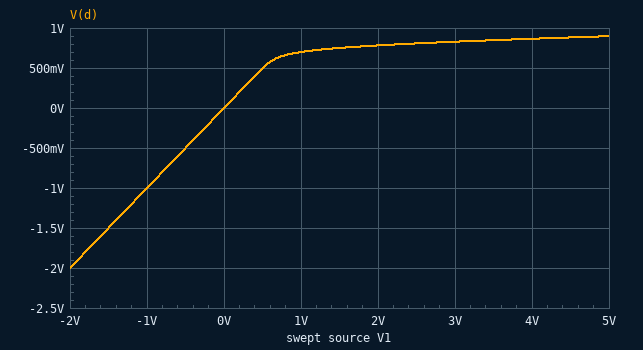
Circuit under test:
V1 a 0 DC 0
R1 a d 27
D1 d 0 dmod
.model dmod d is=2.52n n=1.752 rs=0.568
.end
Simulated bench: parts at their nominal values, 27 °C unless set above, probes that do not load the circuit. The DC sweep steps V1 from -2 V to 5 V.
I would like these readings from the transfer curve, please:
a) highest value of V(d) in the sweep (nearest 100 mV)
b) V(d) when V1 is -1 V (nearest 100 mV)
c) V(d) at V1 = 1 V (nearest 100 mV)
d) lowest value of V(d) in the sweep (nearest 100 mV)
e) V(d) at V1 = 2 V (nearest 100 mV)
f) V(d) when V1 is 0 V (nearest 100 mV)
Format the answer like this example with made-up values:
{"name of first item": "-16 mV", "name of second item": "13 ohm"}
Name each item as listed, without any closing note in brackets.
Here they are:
{"highest value of V(d) in the sweep": "900 mV", "V(d) when V1 is -1 V": "-1.0 V", "V(d) at V1 = 1 V": "700 mV", "lowest value of V(d) in the sweep": "-2.0 V", "V(d) at V1 = 2 V": "800 mV", "V(d) when V1 is 0 V": "0 V"}
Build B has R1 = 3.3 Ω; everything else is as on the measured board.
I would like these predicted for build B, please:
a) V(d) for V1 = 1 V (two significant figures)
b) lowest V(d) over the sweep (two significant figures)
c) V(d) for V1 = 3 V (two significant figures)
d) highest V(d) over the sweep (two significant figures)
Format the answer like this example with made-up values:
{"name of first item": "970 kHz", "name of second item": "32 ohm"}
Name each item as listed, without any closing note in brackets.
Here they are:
{"V(d) for V1 = 1 V": "800 mV", "lowest V(d) over the sweep": "-2.0 V", "V(d) for V1 = 3 V": "1.2 V", "highest V(d) over the sweep": "1.5 V"}
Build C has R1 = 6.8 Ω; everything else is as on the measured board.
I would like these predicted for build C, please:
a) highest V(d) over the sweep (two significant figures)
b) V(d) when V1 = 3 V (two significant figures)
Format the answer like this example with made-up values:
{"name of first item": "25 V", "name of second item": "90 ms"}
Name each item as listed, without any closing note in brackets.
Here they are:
{"highest V(d) over the sweep": "1.2 V", "V(d) when V1 = 3 V": "1.0 V"}
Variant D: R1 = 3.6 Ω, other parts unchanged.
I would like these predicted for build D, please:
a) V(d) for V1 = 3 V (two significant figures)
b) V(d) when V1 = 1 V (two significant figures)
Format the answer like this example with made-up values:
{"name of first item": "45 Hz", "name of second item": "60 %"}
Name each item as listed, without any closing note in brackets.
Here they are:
{"V(d) for V1 = 3 V": "1.2 V", "V(d) when V1 = 1 V": "800 mV"}
